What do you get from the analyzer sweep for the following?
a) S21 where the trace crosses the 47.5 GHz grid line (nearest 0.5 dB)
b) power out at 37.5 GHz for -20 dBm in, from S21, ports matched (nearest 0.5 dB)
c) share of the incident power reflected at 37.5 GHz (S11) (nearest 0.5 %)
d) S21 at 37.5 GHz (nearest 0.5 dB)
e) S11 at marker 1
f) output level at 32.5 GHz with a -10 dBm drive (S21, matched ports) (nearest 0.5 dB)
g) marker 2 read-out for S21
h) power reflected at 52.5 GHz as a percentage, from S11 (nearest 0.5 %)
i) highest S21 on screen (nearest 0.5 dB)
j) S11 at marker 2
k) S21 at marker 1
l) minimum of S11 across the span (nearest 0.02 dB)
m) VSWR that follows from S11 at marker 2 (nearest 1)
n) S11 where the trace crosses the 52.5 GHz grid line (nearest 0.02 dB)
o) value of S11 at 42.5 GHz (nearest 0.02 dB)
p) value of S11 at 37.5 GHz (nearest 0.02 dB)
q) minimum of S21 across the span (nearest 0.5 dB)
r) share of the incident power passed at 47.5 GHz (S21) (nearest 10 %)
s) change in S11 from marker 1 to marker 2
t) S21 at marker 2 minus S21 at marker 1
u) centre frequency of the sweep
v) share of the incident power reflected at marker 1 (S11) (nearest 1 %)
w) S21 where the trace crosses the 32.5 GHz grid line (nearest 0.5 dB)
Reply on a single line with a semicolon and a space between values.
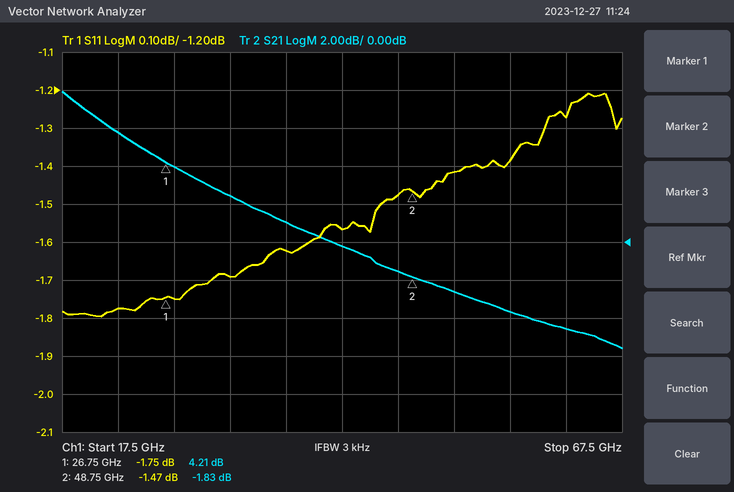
-1.5 dB; -19.0 dBm; 69.0 %; 1.0 dB; -1.75 dB; -7.5 dBm; -1.83 dB; 72.0 %; 8.0 dB; -1.47 dB; 4.21 dB; -1.80 dB; 12; -1.42 dB; -1.56 dB; -1.62 dB; -5.5 dB; 70 %; 0.28 dB; -6.04 dB; 42.5 GHz; 67 %; 2.5 dB
